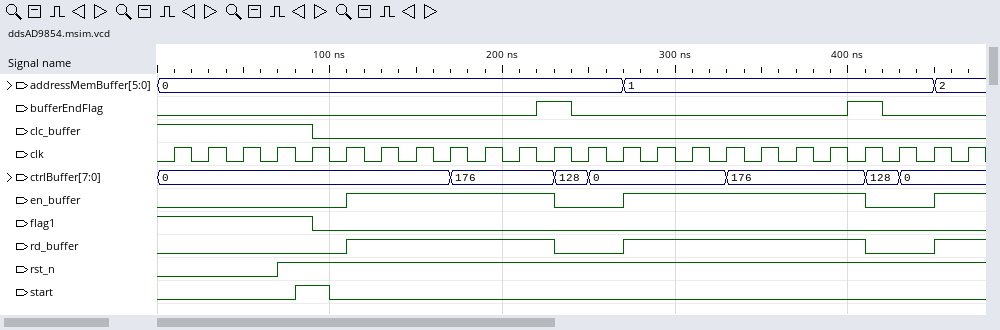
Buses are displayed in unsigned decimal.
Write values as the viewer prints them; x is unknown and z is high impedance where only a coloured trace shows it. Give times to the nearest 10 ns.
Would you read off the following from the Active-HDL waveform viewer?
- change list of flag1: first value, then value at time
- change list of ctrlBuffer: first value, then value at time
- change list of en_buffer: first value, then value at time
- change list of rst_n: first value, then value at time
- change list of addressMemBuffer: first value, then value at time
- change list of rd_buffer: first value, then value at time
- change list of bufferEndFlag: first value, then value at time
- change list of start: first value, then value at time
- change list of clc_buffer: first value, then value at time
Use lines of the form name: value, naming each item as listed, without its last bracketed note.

change list of flag1: first value, then value at time: 1, 0 at 90 ns
change list of ctrlBuffer: first value, then value at time: 0, 176 at 170 ns, 128 at 230 ns, 0 at 250 ns, 176 at 330 ns, 128 at 410 ns, 0 at 430 ns
change list of en_buffer: first value, then value at time: 0, 1 at 110 ns, 0 at 230 ns, 1 at 270 ns, 0 at 410 ns, 1 at 450 ns
change list of rst_n: first value, then value at time: 0, 1 at 70 ns
change list of addressMemBuffer: first value, then value at time: 0, 1 at 270 ns, 2 at 450 ns
change list of rd_buffer: first value, then value at time: 0, 1 at 110 ns, 0 at 230 ns, 1 at 270 ns, 0 at 410 ns, 1 at 450 ns
change list of bufferEndFlag: first value, then value at time: 0, 1 at 220 ns, 0 at 240 ns, 1 at 400 ns, 0 at 420 ns
change list of start: first value, then value at time: 0, 1 at 80 ns, 0 at 100 ns
change list of clc_buffer: first value, then value at time: 1, 0 at 90 ns
